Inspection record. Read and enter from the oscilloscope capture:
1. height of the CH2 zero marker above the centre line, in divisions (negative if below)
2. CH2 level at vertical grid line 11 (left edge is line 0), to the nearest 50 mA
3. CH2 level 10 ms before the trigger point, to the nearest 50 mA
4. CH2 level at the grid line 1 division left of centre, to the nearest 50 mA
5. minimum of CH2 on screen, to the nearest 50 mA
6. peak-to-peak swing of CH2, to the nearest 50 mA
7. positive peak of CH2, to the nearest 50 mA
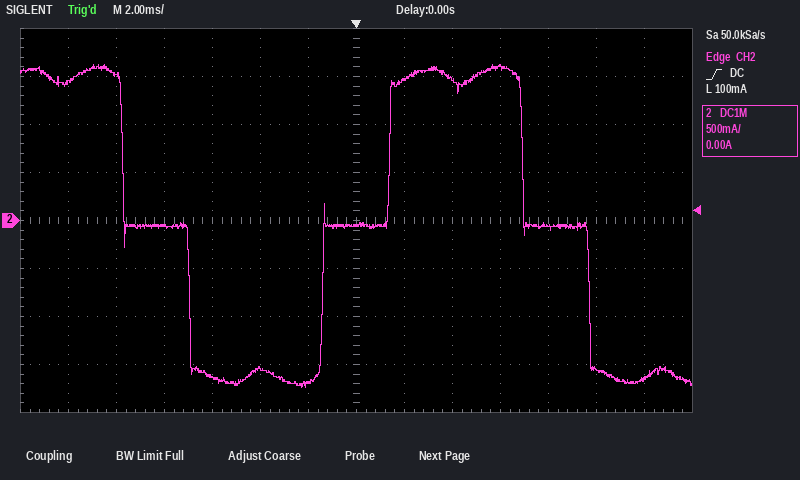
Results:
0.0 div
-50 mA
1.50 A
-1.70 A
-1.75 A
3.35 A
1.60 A
